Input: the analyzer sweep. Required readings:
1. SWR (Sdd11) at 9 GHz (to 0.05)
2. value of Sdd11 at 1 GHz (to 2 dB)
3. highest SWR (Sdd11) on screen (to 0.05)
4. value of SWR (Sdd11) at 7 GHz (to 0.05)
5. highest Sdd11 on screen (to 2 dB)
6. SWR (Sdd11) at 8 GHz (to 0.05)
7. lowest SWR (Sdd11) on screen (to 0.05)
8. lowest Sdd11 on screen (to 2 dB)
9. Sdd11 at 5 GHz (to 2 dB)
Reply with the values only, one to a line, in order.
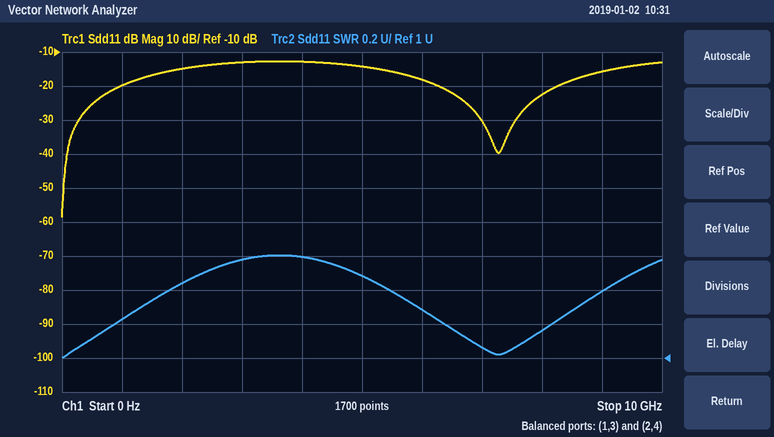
1.40
-20 dB
1.60
1.05
-12 dB
1.15
1.00
-58 dB
-14 dB
